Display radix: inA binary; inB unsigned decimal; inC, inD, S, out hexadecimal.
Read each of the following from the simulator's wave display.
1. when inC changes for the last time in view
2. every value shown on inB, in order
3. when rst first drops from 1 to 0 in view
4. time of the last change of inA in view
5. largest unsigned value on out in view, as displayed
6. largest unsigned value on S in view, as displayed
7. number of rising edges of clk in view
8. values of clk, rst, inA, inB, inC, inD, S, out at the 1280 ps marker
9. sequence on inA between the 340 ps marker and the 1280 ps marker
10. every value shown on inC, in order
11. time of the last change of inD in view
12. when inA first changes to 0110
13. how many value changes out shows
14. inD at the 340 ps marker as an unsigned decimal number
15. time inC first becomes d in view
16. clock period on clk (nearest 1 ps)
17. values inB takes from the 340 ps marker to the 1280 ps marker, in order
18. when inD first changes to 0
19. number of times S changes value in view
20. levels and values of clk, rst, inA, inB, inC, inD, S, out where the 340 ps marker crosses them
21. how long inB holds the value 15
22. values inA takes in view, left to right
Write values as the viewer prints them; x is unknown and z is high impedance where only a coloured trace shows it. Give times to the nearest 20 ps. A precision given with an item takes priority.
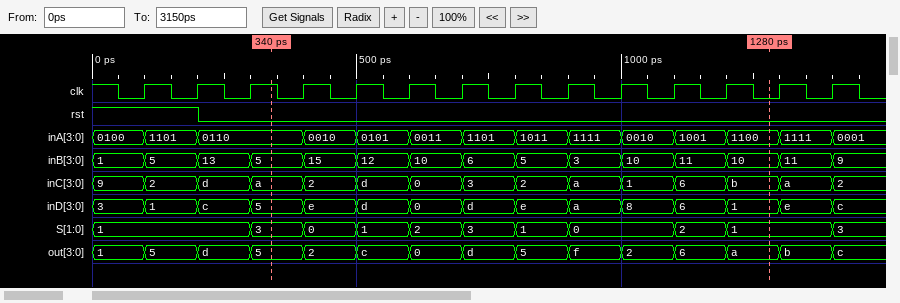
1400 ps
1, 5, 13, 5, 15, 12, 10, 6, 5, 3, 10, 11, 10, 11, 9
200 ps
1400 ps
f
3
14
clk=0, rst=0, inA=1100, inB=10, inC=b, inD=1, S=1, out=a
0110, 0010, 0101, 0011, 1101, 1011, 1111, 0010, 1001, 1100
9, 2, d, a, 2, d, 0, 3, 2, a, 1, 6, b, a, 2
1400 ps
200 ps
14
5
200 ps
100 ps
5, 15, 12, 10, 6, 5, 3, 10, 11, 10
600 ps
10
clk=1, rst=0, inA=0110, inB=5, inC=a, inD=5, S=3, out=5
100 ps
0100, 1101, 0110, 0010, 0101, 0011, 1101, 1011, 1111, 0010, 1001, 1100, 1111, 0001
